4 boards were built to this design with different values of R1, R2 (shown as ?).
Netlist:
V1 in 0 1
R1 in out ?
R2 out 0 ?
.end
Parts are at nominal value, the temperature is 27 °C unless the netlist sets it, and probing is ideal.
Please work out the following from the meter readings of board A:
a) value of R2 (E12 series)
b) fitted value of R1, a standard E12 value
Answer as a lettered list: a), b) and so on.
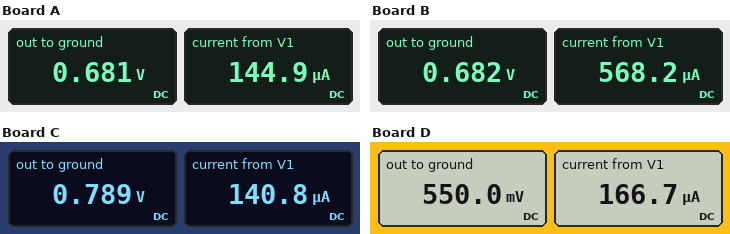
a) 4.7 kΩ
b) 2.2 kΩ
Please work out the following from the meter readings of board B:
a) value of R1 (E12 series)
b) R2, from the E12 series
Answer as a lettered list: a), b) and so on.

a) 560 Ω
b) 1.2 kΩ
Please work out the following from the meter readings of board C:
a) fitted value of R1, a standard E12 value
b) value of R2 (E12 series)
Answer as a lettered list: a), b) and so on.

a) 1.5 kΩ
b) 5.6 kΩ
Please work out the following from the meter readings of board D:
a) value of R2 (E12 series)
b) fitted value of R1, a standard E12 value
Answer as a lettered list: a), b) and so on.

a) 3.3 kΩ
b) 2.7 kΩ
